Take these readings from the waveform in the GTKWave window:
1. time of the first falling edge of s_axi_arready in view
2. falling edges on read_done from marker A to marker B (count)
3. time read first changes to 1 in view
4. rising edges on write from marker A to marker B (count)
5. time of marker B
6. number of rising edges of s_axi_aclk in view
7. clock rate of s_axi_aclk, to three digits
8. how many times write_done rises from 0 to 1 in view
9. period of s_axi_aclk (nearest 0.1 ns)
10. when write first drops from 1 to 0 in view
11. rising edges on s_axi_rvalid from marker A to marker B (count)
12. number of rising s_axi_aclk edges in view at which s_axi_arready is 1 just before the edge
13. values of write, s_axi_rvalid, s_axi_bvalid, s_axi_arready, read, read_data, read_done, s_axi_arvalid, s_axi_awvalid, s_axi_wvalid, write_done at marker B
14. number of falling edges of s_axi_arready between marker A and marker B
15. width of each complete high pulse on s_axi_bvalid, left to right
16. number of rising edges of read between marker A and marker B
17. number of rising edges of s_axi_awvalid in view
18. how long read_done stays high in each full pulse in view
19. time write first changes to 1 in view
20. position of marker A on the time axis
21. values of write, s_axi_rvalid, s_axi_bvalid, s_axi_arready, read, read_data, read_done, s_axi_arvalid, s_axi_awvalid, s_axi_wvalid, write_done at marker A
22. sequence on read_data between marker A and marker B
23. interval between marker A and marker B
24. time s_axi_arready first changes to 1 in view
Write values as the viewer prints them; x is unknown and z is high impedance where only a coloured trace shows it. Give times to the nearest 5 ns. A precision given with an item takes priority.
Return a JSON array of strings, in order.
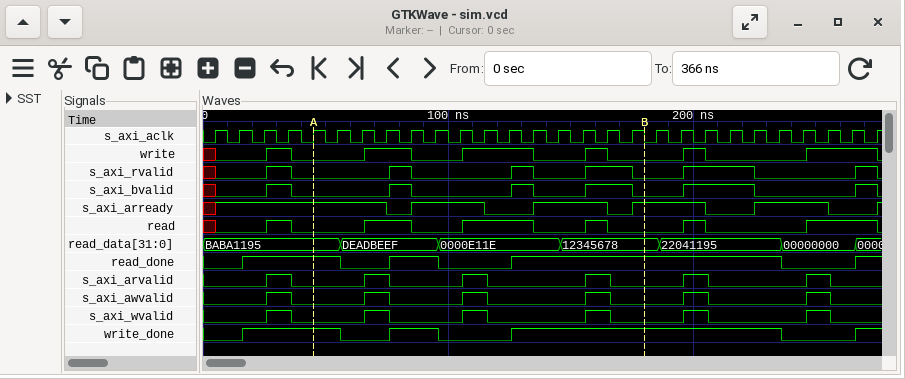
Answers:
["75 ns", "2", "25 ns", "3", "180 ns", "28", "100 MHz", "4", "10 ns", "35 ns", "3", "19", "write=0, s_axi_rvalid=0, s_axi_bvalid=0, s_axi_arready=1, read=0, read_data=12345678, read_done=1, s_axi_arvalid=0, s_axi_awvalid=0, s_axi_wvalid=0, write_done=1", "3", "10 ns, 10 ns, 10 ns, 20 ns, 30 ns, 10 ns", "3", "6", "40 ns, 20 ns, 110 ns", "25 ns", "45 ns", "write=0, s_axi_rvalid=0, s_axi_bvalid=0, s_axi_arready=1, read=0, read_data=BABA1195, read_done=1, s_axi_arvalid=0, s_axi_awvalid=0, s_axi_wvalid=0, write_done=1", "BABA1195, DEADBEEF, 0000E11E, 12345678", "135 ns", "5 ns"]
